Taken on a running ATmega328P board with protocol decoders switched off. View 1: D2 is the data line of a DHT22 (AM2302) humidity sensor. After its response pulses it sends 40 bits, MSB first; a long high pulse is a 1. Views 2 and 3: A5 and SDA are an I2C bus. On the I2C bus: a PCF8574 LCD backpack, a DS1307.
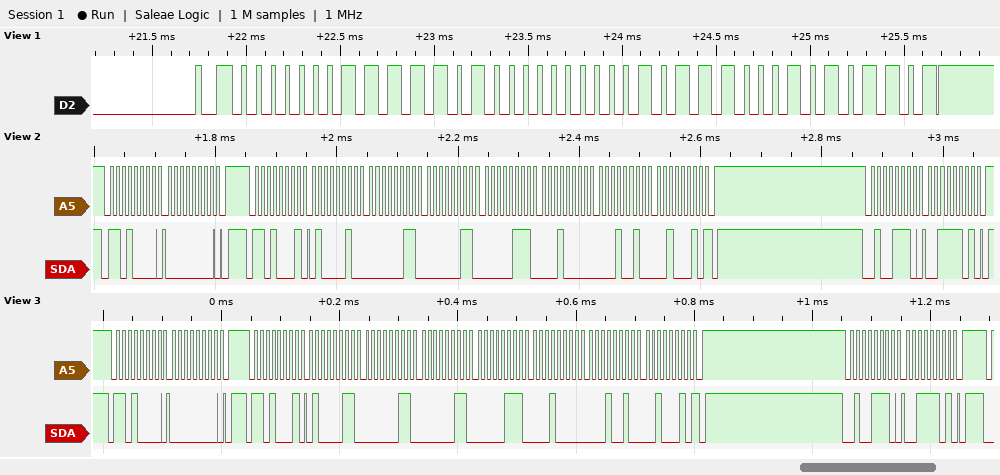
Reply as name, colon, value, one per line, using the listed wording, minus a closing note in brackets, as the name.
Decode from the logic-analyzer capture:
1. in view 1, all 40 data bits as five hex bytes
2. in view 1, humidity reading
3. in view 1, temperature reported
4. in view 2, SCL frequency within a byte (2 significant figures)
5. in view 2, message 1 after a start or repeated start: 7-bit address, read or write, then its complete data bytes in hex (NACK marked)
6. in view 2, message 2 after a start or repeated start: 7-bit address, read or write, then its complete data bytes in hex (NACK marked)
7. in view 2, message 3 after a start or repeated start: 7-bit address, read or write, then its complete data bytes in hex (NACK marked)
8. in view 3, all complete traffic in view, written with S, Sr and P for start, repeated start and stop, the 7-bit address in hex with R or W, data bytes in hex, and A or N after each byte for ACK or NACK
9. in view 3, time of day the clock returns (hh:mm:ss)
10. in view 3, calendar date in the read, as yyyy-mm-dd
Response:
in view 1, all 40 data bits as five hex bytes: 01 F4 00 B8 AD
in view 1, humidity reading: 50.0 %
in view 1, temperature reported: 18.4 °C
in view 2, SCL frequency within a byte: 100 kHz
in view 2, message 1 after a start or repeated start: 7-bit address, read or write, then its complete data bytes in hex: 0x68 write: 00
in view 2, message 2 after a start or repeated start: 7-bit address, read or write, then its complete data bytes in hex: 0x68 read: 42 03 03 07 10 12 22 NACK
in view 2, message 3 after a start or repeated start: 7-bit address, read or write, then its complete data bytes in hex: 0x27 write: 3D
in view 3, all complete traffic in view, written with S, Sr and P for start, repeated start and stop, the 7-bit address in hex with R or W, data bytes in hex, and A or N after each byte for ACK or NACK: S 68W A 00 A P S 68R A 43 A 03 A 03 A 07 A 10 A 12 A 22 N P S 27W A 3D A P
in view 3, time of day the clock returns: 03:03:43
in view 3, calendar date in the read, as yyyy-mm-dd: 2022-12-10
